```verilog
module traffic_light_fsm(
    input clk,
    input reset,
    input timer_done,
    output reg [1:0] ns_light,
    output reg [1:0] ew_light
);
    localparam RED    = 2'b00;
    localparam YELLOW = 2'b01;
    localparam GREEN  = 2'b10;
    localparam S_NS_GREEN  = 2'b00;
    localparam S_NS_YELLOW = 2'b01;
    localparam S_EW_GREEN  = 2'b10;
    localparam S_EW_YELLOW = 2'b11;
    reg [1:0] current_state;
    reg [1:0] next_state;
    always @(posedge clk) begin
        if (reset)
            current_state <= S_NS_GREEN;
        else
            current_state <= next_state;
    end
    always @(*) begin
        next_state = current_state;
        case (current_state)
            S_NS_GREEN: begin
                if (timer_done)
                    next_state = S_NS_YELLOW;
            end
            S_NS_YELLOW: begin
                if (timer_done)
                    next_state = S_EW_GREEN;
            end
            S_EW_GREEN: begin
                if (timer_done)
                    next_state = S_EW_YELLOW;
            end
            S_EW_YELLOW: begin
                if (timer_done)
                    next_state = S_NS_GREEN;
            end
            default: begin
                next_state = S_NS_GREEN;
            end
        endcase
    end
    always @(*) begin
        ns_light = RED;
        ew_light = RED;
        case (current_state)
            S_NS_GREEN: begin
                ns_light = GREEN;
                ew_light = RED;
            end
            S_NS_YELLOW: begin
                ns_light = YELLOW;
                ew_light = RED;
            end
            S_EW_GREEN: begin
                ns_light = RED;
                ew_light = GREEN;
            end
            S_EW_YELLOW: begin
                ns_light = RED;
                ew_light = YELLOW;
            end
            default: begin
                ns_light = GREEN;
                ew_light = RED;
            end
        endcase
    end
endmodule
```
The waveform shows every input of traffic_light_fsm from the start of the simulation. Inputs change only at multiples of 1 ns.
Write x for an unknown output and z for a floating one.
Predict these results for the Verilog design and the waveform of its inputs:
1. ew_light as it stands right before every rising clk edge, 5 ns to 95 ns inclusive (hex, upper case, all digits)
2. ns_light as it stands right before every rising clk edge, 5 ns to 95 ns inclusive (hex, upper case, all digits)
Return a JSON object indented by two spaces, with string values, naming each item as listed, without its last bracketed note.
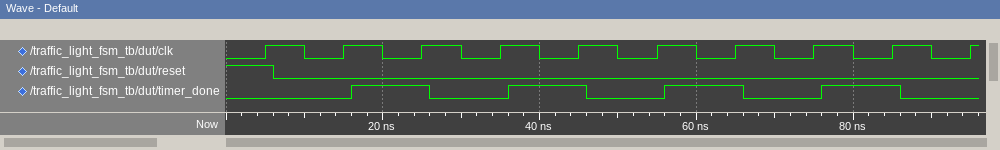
{
  "ew_light as it stands right before every rising clk edge, 5 ns to 95 ns inclusive": "x, 0, 0, 0, 0, 2, 2, 1, 1, 0",
  "ns_light as it stands right before every rising clk edge, 5 ns to 95 ns inclusive": "x, 2, 2, 1, 1, 0, 0, 0, 0, 2"
}
